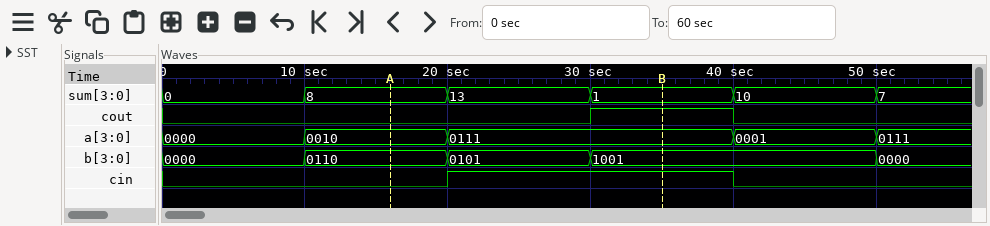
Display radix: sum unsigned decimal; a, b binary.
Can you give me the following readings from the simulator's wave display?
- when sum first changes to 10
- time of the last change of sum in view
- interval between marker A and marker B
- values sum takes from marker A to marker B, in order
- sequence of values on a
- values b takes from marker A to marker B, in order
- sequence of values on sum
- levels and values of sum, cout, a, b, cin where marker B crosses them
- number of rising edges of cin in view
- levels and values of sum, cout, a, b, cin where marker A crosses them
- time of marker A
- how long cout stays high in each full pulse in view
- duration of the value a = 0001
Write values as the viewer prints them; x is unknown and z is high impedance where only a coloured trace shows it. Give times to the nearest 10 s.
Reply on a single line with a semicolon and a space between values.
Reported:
40 s; 50 s; 20 s; 8, 13, 1; 0000, 0010, 0111, 0001, 0111; 0110, 0101, 1001; 0, 8, 13, 1, 10, 7; sum=1, cout=1, a=0111, b=1001, cin=1; 1; sum=8, cout=0, a=0010, b=0110, cin=0; 20 s; 10 s; 10 s
